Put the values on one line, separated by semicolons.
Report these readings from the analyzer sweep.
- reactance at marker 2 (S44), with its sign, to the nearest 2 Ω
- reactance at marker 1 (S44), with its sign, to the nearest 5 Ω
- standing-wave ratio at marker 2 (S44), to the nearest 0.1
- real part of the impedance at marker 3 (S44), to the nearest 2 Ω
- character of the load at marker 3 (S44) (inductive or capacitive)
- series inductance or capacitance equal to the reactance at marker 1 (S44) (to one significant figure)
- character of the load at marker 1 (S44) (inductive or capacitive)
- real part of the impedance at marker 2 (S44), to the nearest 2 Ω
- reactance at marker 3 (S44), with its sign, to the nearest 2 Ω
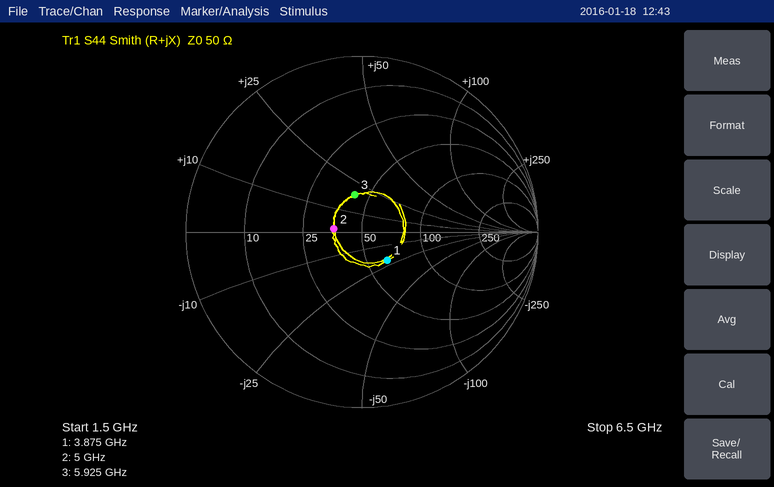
+2 Ω; -20 Ω; 1.4; 42 Ω; inductive; 2 pF; capacitive; 36 Ω; +18 Ω
